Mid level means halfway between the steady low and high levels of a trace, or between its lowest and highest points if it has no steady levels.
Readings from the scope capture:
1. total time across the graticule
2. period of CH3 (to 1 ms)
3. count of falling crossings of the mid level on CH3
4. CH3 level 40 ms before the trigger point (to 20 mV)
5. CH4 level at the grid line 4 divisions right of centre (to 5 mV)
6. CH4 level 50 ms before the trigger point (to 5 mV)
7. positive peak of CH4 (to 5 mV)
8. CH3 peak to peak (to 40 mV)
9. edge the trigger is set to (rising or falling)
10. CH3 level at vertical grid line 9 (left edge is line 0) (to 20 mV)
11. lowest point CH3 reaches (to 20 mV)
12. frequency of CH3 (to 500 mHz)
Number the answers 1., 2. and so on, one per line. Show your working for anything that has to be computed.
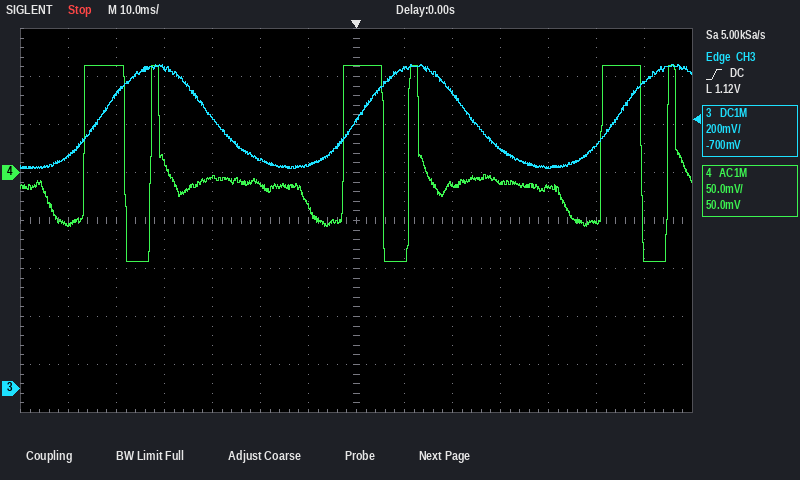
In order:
1. 140 ms
2. 54 ms
3. 2
4. 1.34 V
5. -15 mV
6. 110 mV
7. 110 mV
8. 440 mV
9. rising
10. 1.24 V
11. 920 mV
12. 1 / 54 ms ≈ 18.5 Hz
